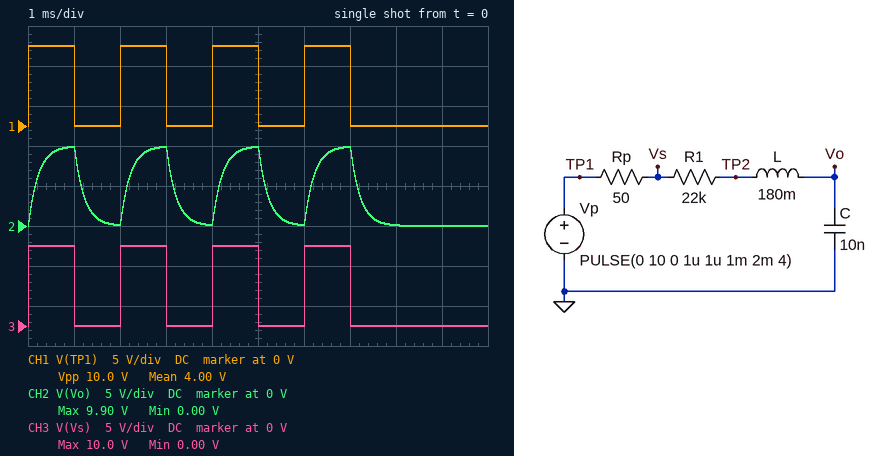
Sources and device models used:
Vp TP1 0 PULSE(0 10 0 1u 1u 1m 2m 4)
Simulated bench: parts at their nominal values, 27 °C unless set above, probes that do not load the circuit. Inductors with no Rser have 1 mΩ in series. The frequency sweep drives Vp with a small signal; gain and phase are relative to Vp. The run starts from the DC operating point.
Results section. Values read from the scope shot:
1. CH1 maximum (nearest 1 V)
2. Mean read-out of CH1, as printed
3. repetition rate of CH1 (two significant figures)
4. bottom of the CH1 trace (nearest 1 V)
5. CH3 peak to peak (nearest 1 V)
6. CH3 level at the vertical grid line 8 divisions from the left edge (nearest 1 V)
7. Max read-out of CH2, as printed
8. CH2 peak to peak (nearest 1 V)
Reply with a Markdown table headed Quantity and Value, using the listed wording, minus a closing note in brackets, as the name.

| Quantity | Value |
|---|---|
| CH1 maximum | 10 V |
| Mean read-out of CH1, as printed | 4.00 V |
| repetition rate of CH1 | 500 Hz |
| bottom of the CH1 trace | 0 V |
| CH3 peak to peak | 10 V |
| CH3 level at the vertical grid line 8 divisions from the left edge | 0 V |
| Max read-out of CH2, as printed | 9.90 V |
| CH2 peak to peak | 10 V |
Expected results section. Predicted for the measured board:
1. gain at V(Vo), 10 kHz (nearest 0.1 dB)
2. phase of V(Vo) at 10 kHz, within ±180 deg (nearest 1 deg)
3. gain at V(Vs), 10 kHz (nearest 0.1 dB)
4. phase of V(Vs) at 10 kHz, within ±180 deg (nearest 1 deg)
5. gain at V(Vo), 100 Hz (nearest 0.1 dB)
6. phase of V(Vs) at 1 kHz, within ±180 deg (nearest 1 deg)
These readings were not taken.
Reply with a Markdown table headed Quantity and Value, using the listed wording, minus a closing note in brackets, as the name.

| Quantity | Value |
|---|---|
| gain at V(Vo), 10 kHz | -23.6 dB |
| phase of V(Vo) at 10 kHz, within ±180 deg | -114 deg |
| gain at V(Vs), 10 kHz | 0 dB |
| phase of V(Vs) at 10 kHz, within ±180 deg | 0 deg |
| gain at V(Vo), 100 Hz | -0.1 dB |
| phase of V(Vs) at 1 kHz, within ±180 deg | 0 deg |
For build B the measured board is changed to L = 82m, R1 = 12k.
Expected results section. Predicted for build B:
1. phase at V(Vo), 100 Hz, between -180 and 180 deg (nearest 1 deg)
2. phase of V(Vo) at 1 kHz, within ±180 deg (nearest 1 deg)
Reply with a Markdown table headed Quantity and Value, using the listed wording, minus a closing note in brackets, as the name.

| Quantity | Value |
|---|---|
| phase at V(Vo), 100 Hz, between -180 and 180 deg | -4 deg |
| phase of V(Vo) at 1 kHz, within ±180 deg | -38 deg |
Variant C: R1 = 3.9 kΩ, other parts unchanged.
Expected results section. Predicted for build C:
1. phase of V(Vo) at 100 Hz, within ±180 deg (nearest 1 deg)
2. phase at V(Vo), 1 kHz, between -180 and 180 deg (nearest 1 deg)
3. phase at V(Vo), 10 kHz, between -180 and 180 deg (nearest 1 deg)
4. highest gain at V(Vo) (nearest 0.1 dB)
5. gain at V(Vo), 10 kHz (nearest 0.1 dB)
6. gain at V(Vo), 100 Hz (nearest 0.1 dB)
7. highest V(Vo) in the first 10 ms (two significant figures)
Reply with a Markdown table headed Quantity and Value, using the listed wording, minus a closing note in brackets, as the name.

| Quantity | Value |
|---|---|
| phase of V(Vo) at 100 Hz, within ±180 deg | -1 deg |
| phase at V(Vo), 1 kHz, between -180 and 180 deg | -15 deg |
| phase at V(Vo), 10 kHz, between -180 and 180 deg | -158 deg |
| highest gain at V(Vo) | 1.7 dB |
| gain at V(Vo), 10 kHz | -16.4 dB |
| gain at V(Vo), 100 Hz | 0 dB |
| highest V(Vo) in the first 10 ms | 12 V |
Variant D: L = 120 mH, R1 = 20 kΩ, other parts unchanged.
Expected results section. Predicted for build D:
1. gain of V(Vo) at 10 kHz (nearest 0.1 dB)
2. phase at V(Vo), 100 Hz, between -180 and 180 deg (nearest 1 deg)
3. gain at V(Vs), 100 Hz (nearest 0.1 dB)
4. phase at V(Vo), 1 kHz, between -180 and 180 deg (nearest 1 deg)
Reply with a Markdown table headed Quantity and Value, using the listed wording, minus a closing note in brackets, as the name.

| Quantity | Value |
|---|---|
| gain of V(Vo) at 10 kHz | -22.4 dB |
| phase at V(Vo), 100 Hz, between -180 and 180 deg | -7 deg |
| gain at V(Vs), 100 Hz | 0 dB |
| phase at V(Vo), 1 kHz, between -180 and 180 deg | -53 deg |
